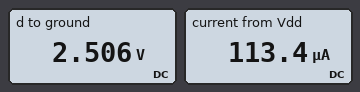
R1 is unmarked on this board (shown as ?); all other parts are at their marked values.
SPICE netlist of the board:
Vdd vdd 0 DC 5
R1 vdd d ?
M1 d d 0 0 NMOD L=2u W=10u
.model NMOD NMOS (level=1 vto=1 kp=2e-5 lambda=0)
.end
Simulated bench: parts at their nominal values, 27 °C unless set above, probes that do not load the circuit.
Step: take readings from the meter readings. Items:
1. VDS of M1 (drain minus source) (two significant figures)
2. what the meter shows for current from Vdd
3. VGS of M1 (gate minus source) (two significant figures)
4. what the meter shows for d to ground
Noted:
2.5 V
113.4 µA
2.5 V
2.506 V
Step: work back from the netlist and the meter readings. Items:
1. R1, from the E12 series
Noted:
22 kΩ
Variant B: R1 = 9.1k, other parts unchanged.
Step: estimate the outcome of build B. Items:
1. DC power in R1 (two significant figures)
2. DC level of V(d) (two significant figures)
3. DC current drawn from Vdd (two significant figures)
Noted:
410 µW
3.1 V
210 µA
